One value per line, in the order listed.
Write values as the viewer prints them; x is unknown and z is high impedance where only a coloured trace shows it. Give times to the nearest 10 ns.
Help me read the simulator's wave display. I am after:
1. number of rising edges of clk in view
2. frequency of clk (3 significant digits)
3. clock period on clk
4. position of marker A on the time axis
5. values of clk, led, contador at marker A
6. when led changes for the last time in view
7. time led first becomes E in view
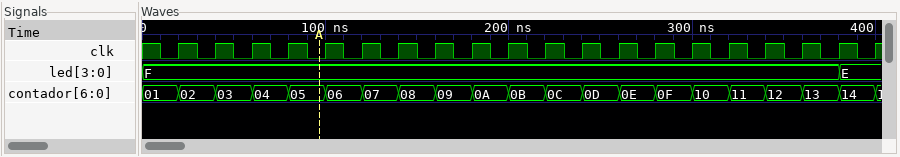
20
50.0 MHz
20 ns
100 ns
clk=0, led=F, contador=05
380 ns
380 ns
